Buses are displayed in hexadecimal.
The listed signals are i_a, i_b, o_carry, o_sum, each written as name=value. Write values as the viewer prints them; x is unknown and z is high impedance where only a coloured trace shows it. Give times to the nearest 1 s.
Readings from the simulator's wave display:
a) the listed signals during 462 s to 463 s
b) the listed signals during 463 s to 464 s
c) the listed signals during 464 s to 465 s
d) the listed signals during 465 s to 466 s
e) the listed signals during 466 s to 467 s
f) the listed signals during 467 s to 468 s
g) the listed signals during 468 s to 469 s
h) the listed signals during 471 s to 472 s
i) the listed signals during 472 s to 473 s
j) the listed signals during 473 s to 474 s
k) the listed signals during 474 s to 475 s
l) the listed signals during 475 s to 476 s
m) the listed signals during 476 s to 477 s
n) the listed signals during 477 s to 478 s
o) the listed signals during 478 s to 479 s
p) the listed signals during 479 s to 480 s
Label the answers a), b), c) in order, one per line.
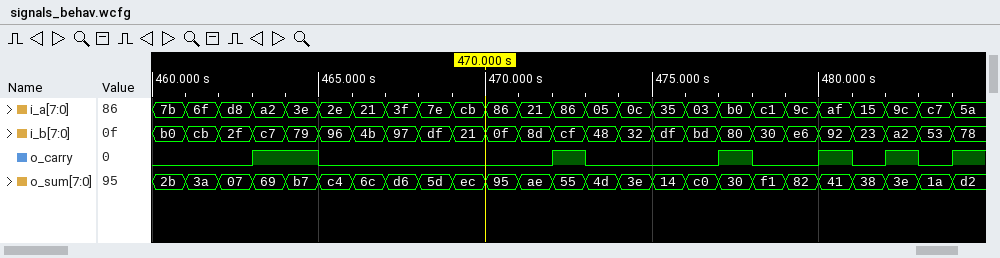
a) i_a=d8, i_b=2f, o_carry=0, o_sum=07
b) i_a=a2, i_b=c7, o_carry=1, o_sum=69
c) i_a=3e, i_b=79, o_carry=1, o_sum=b7
d) i_a=2e, i_b=96, o_carry=0, o_sum=c4
e) i_a=21, i_b=4b, o_carry=0, o_sum=6c
f) i_a=3f, i_b=97, o_carry=0, o_sum=d6
g) i_a=7e, i_b=df, o_carry=0, o_sum=5d
h) i_a=21, i_b=8d, o_carry=0, o_sum=ae
i) i_a=86, i_b=cf, o_carry=1, o_sum=55
j) i_a=05, i_b=48, o_carry=0, o_sum=4d
k) i_a=0c, i_b=32, o_carry=0, o_sum=3e
l) i_a=35, i_b=df, o_carry=0, o_sum=14
m) i_a=03, i_b=bd, o_carry=0, o_sum=c0
n) i_a=b0, i_b=80, o_carry=1, o_sum=30
o) i_a=c1, i_b=30, o_carry=0, o_sum=f1
p) i_a=9c, i_b=e6, o_carry=0, o_sum=82
